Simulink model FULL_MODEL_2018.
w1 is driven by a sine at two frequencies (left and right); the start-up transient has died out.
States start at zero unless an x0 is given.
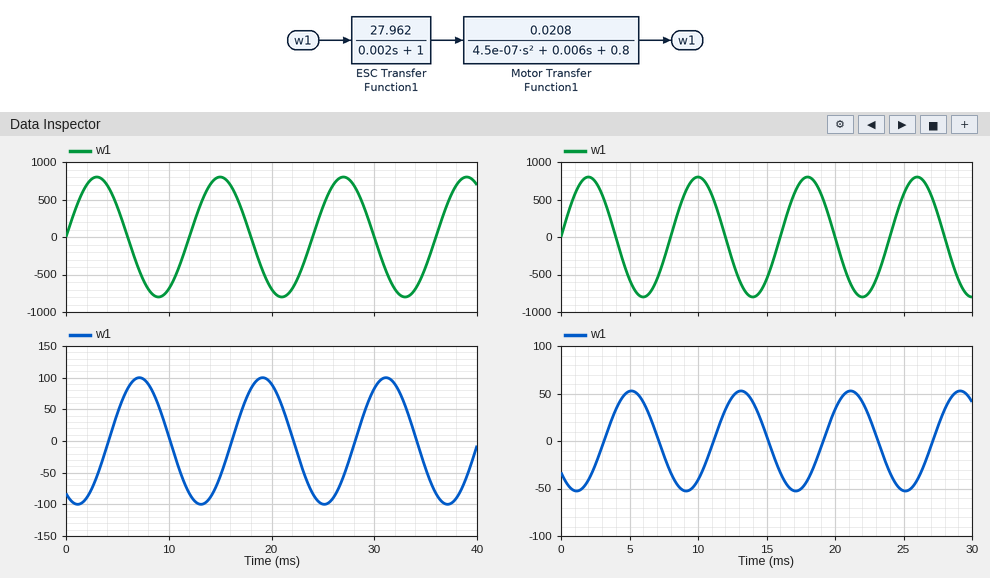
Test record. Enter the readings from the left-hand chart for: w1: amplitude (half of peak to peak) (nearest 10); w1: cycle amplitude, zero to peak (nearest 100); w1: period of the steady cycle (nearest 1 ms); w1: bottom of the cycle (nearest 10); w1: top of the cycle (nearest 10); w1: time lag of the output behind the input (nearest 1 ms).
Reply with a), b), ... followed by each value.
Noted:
a) 100
b) 800
c) 12 ms
d) -100
e) 100
f) 4 ms
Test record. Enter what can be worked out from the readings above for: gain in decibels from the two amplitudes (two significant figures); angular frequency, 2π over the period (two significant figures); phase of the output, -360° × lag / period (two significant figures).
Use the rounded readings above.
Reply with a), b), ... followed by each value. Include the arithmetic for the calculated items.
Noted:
a) 20 log10(100 / 800) = -18 dB
b) 2π / 12 = 0.52 rad/ms
c) -360 × 4 / 12 = -120°
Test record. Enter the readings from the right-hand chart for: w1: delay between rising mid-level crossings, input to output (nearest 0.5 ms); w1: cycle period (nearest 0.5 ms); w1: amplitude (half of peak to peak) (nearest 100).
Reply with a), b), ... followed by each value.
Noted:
a) 3.0 ms
b) 8.0 ms
c) 800
